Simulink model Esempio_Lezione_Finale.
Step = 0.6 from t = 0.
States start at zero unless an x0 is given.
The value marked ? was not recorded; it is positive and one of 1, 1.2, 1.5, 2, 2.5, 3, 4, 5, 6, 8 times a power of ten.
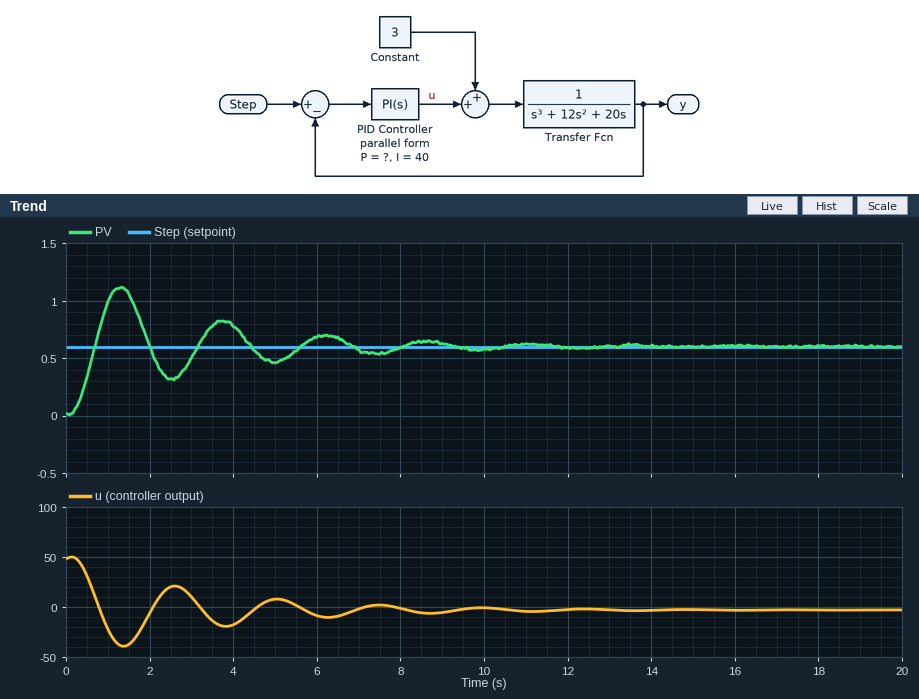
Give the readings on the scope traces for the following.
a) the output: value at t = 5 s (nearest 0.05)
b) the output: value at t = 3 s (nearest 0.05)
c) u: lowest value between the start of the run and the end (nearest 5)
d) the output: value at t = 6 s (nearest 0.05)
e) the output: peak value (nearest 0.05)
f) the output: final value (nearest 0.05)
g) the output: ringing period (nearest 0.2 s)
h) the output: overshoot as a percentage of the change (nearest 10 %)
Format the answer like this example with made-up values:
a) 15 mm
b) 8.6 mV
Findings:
a) 0.45
b) 0.50
c) -40
d) 0.70
e) 1.10
f) 0.60
g) 2.4 s
h) 90 %
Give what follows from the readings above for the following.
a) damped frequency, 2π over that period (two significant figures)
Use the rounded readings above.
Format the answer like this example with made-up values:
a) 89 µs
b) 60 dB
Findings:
a) 2.6 rad/s
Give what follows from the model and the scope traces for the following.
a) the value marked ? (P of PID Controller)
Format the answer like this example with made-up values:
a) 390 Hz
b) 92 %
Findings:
a) 80
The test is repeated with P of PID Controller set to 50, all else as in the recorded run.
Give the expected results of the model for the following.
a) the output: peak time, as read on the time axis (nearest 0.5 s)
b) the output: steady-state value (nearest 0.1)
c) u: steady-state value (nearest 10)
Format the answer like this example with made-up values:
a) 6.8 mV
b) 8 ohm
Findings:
a) 1.5 s
b) 0.6
c) 0
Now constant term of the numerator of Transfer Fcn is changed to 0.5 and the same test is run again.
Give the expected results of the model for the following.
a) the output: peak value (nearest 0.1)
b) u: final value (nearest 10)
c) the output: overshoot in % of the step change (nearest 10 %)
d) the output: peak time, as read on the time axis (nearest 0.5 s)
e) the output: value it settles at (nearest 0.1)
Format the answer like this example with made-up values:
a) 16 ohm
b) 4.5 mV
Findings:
a) 1.0
b) 0
c) 70 %
d) 2.0 s
e) 0.6
